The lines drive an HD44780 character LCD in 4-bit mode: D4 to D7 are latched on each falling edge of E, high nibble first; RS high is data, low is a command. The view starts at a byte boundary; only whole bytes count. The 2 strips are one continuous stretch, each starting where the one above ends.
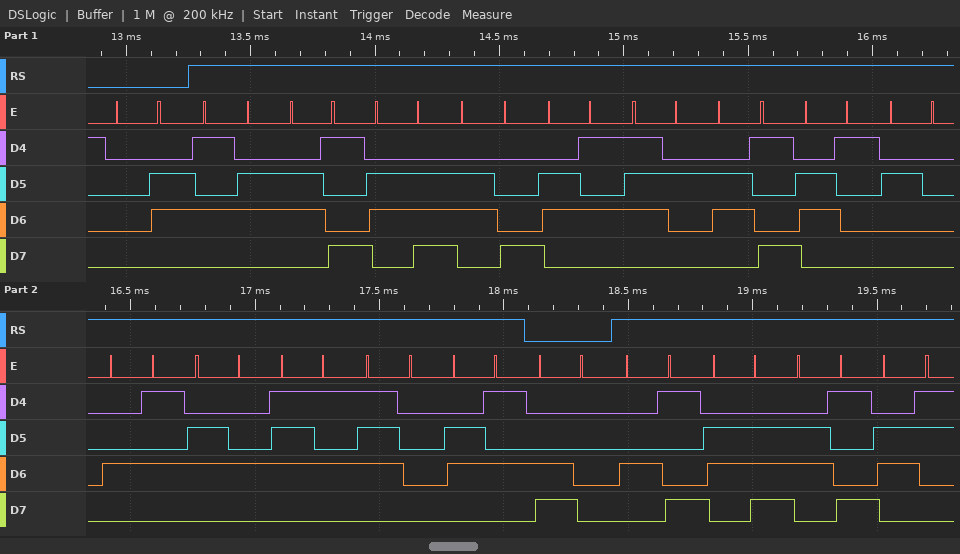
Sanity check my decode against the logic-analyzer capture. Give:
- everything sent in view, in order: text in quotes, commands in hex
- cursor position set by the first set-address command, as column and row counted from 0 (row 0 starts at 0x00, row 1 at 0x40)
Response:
0x06 "Vinheria Edupe" 0xC0 "Inic"
column 0, row 1
